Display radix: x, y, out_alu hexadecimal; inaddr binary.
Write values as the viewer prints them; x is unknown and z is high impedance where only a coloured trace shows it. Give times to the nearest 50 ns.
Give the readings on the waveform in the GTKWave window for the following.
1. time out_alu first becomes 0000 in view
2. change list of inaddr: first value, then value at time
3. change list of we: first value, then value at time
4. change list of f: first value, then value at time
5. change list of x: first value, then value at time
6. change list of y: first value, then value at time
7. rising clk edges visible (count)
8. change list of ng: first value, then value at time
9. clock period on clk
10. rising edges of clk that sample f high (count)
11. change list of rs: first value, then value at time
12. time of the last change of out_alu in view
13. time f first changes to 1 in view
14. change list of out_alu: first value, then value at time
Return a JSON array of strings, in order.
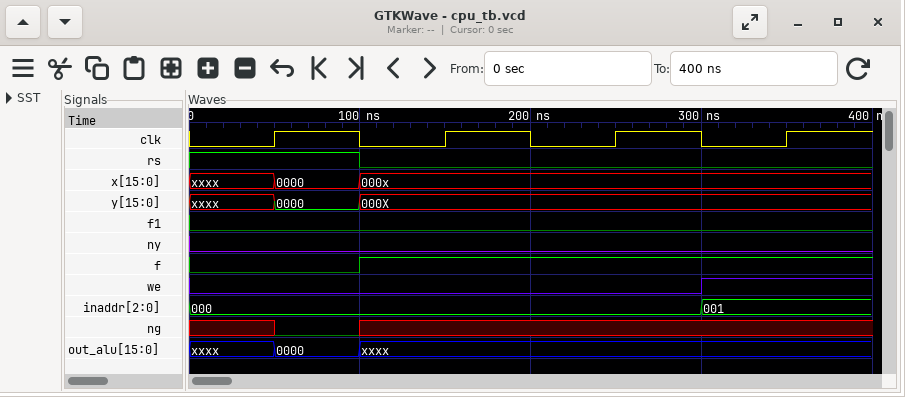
["50 ns", "000, 001 at 300 ns", "0, 1 at 300 ns", "0, 1 at 100 ns", "xxxx, 0000 at 50 ns, 000x at 100 ns", "xxxx, 0000 at 50 ns, 000X at 100 ns", "4", "x, 0 at 50 ns, x at 100 ns", "100 ns", "3", "1, 0 at 100 ns", "100 ns", "100 ns", "xxxx, 0000 at 50 ns, xxxx at 100 ns"]
